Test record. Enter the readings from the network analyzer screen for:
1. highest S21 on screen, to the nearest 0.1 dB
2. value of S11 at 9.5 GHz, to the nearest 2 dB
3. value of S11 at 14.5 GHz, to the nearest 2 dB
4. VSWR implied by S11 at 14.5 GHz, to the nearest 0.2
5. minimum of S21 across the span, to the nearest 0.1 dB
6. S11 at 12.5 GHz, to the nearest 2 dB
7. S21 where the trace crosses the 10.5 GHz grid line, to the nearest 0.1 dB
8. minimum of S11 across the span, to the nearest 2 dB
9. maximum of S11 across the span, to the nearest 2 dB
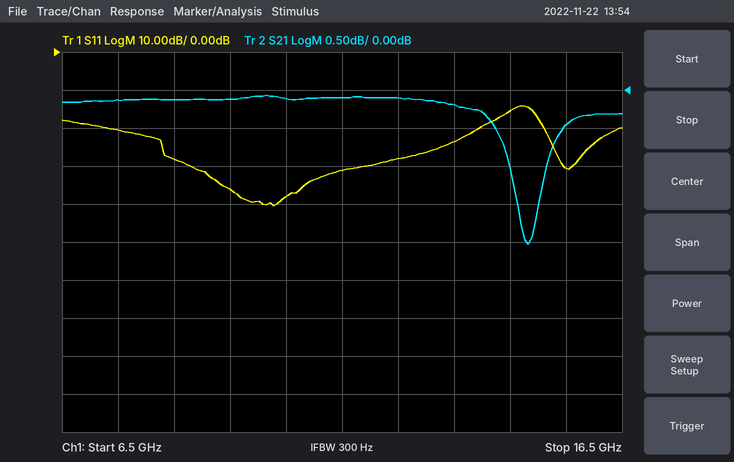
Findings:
-0.1 dB
-36 dB
-16 dB
1.4
-2.0 dB
-28 dB
-0.1 dB
-40 dB
-14 dB
